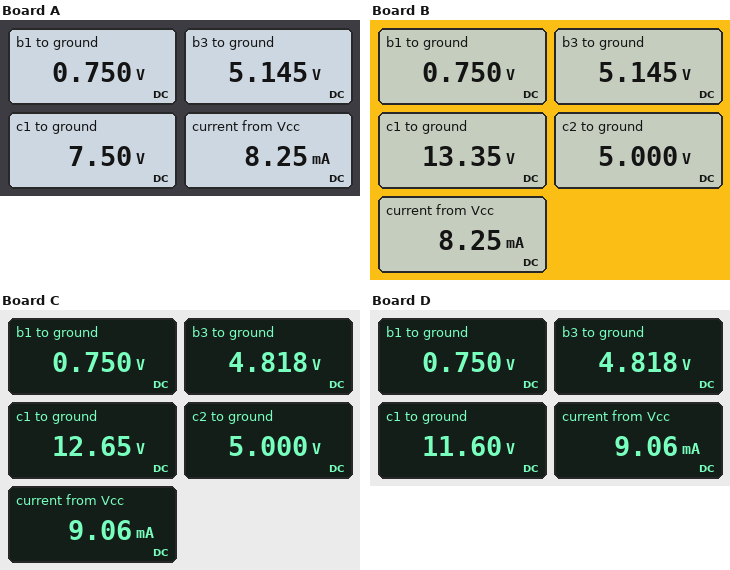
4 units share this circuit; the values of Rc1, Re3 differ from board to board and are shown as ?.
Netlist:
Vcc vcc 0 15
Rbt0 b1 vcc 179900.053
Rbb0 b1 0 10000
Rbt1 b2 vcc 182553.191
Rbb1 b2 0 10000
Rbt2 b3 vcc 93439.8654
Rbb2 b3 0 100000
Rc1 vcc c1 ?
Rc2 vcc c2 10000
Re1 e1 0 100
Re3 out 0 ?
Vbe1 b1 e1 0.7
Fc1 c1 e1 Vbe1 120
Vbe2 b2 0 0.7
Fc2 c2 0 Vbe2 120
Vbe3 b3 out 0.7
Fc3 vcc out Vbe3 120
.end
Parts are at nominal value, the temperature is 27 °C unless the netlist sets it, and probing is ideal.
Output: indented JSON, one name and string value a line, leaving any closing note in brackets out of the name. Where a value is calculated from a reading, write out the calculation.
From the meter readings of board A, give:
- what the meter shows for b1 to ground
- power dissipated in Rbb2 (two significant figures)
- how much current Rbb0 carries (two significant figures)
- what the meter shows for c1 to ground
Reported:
{
  "what the meter shows for b1 to ground": "0.750 V",
  "power dissipated in Rbb2": "(5.145 V)^2 / 100 kΩ = 260 µW",
  "how much current Rbb0 carries": "(750 mV) / 10 kΩ = 75 µA",
  "what the meter shows for c1 to ground": "7.50 V"
}
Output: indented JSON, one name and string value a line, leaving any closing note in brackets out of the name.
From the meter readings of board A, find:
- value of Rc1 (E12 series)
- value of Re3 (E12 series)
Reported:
{
  "value of Rc1": "15 kΩ",
  "value of Re3": "680 Ω"
}
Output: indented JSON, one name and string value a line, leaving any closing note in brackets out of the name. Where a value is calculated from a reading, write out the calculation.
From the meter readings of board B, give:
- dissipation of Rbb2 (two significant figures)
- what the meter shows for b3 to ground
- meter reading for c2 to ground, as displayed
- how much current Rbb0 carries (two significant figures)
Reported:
{
  "dissipation of Rbb2": "(5.145 V)^2 / 100 kΩ = 260 µW",
  "what the meter shows for b3 to ground": "5.145 V",
  "meter reading for c2 to ground, as displayed": "5.000 V",
  "how much current Rbb0 carries": "(750 mV) / 10 kΩ = 75 µA"
}
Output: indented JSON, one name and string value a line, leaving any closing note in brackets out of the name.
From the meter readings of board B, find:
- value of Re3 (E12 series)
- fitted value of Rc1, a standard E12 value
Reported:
{
  "value of Re3": "680 Ω",
  "fitted value of Rc1, a standard E12 value": "3.3 kΩ"
}
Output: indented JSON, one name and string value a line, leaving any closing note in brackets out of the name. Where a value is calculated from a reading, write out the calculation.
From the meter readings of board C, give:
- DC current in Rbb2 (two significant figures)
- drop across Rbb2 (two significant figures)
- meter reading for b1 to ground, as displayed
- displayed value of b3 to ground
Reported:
{
  "DC current in Rbb2": "(4.818 V) / 100 kΩ = 48 µA",
  "drop across Rbb2": "4.818 V = 4.8 V",
  "meter reading for b1 to ground, as displayed": "0.750 V",
  "displayed value of b3 to ground": "4.818 V"
}
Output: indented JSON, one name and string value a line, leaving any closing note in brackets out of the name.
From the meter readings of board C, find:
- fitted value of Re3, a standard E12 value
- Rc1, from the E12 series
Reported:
{
  "fitted value of Re3, a standard E12 value": "560 Ω",
  "Rc1, from the E12 series": "4.7 kΩ"
}
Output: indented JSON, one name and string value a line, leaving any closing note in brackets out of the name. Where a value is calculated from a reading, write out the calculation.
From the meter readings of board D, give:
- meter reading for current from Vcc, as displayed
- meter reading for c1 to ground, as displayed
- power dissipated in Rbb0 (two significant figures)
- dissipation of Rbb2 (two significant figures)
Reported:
{
  "meter reading for current from Vcc, as displayed": "9.06 mA",
  "meter reading for c1 to ground, as displayed": "11.60 V",
  "power dissipated in Rbb0": "(750 mV)^2 / 10 kΩ = 56 µW",
  "dissipation of Rbb2": "(4.818 V)^2 / 100 kΩ = 230 µW"
}
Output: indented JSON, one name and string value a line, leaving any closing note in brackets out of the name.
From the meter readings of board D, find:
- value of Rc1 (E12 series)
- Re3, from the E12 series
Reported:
{
  "value of Rc1": "6.8 kΩ",
  "Re3, from the E12 series": "560 Ω"
}
